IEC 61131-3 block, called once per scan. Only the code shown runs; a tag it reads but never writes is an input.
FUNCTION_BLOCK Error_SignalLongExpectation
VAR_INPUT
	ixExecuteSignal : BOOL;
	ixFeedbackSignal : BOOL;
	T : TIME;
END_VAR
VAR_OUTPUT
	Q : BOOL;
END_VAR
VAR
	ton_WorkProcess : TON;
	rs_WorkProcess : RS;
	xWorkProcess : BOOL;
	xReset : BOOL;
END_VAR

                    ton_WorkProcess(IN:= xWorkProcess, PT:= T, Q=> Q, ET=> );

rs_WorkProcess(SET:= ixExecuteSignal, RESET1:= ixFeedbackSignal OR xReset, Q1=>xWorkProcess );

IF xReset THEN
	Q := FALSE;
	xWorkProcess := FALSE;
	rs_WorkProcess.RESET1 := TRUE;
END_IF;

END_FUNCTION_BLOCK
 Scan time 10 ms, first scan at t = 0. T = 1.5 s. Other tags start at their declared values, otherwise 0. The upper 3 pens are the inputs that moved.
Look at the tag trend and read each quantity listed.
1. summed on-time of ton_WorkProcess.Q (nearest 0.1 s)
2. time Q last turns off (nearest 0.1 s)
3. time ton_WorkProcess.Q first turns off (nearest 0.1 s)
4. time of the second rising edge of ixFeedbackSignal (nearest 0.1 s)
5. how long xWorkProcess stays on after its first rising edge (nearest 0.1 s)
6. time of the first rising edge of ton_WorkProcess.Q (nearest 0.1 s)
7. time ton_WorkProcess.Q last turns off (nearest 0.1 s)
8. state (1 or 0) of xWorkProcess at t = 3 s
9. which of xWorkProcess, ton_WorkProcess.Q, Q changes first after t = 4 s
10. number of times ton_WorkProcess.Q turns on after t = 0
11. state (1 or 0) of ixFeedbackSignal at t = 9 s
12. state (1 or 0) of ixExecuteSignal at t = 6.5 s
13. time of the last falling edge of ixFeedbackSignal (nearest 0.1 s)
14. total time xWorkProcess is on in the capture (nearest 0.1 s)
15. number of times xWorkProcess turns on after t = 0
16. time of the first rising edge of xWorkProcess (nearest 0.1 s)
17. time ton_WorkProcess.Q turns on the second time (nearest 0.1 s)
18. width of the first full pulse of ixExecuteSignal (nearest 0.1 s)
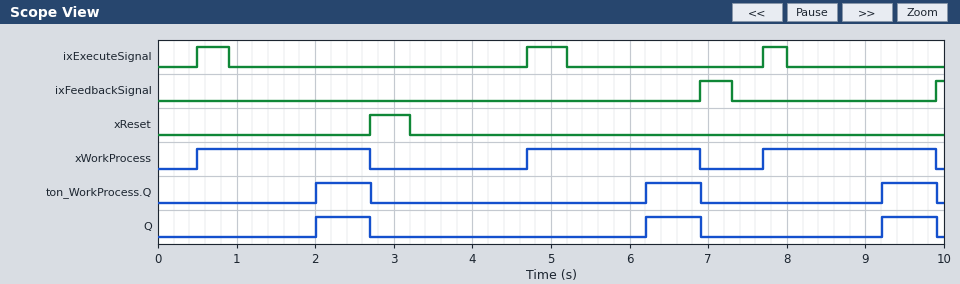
2.1 s
9.9 s
2.7 s
9.9 s
2.2 s
2.0 s
9.9 s
0
xWorkProcess
3
0
0
7.3 s
6.6 s
3
0.5 s
6.2 s
0.4 s
